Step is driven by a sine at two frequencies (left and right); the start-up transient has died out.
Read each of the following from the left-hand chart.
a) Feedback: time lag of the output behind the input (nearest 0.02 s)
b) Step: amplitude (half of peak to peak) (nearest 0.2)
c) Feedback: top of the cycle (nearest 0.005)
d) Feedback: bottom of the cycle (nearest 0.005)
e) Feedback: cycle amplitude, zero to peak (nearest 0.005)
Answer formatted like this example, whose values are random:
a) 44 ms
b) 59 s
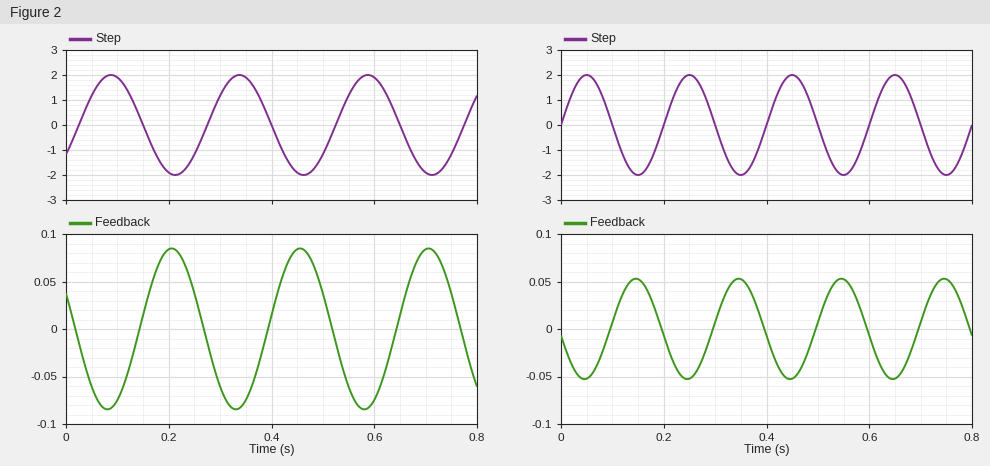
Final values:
a) 0.12 s
b) 2.0
c) 0.085
d) -0.085
e) 0.085
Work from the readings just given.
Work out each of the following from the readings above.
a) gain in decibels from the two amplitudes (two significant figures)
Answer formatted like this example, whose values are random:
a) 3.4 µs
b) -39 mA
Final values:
a) -27 dB
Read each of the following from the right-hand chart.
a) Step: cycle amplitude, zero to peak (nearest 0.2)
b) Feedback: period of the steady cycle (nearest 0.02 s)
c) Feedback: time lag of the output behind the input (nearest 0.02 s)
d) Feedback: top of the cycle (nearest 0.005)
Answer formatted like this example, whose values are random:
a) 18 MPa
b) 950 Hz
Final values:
a) 2.0
b) 0.20 s
c) 0.10 s
d) 0.055
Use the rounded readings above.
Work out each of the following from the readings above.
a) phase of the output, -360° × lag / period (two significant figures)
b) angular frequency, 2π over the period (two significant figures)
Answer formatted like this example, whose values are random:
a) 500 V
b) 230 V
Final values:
a) -180°
b) 31 rad/s
